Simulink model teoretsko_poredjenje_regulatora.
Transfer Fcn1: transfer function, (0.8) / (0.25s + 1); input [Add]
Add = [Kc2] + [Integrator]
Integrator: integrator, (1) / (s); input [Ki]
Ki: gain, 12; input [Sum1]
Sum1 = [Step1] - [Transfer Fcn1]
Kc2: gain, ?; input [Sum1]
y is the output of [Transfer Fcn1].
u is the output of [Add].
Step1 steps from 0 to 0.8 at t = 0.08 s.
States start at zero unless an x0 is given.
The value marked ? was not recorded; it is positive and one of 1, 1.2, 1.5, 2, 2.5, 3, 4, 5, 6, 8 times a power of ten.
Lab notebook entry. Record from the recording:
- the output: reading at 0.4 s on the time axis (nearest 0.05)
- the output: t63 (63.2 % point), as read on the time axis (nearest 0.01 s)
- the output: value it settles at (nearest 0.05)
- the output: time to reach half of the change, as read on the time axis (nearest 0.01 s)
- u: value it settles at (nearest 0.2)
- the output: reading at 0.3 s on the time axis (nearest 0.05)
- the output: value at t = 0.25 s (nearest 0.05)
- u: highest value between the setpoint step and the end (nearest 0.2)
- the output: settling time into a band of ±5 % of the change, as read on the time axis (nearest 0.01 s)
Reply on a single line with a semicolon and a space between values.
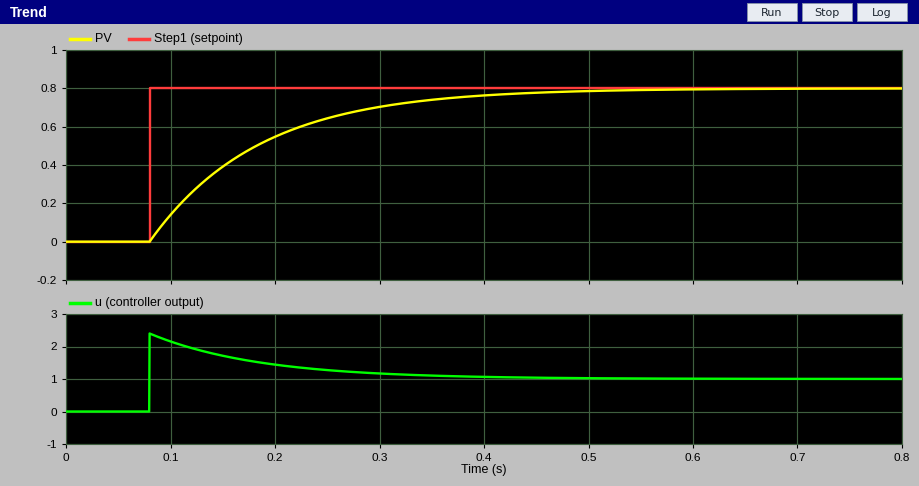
0.75; 0.18 s; 0.80; 0.15 s; 1.0; 0.70; 0.65; 2.4; 0.39 s
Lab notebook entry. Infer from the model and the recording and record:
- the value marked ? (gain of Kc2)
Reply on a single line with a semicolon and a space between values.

3
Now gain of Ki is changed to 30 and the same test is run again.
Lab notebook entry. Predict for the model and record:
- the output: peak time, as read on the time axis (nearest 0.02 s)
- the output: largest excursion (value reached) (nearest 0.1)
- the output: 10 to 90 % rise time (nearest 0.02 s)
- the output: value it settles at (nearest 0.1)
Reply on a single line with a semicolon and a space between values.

0.36 s; 0.9; 0.12 s; 0.8
